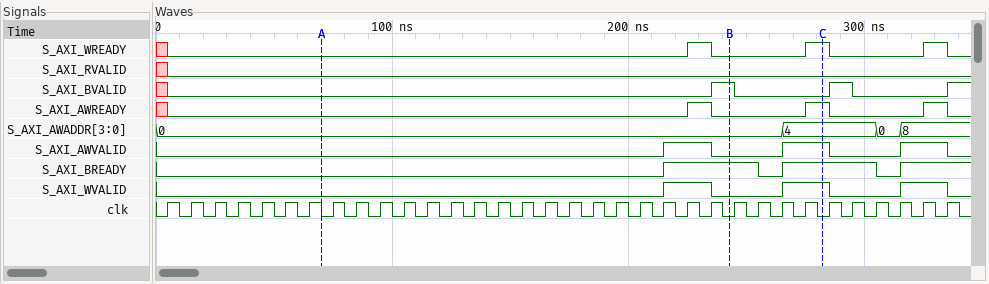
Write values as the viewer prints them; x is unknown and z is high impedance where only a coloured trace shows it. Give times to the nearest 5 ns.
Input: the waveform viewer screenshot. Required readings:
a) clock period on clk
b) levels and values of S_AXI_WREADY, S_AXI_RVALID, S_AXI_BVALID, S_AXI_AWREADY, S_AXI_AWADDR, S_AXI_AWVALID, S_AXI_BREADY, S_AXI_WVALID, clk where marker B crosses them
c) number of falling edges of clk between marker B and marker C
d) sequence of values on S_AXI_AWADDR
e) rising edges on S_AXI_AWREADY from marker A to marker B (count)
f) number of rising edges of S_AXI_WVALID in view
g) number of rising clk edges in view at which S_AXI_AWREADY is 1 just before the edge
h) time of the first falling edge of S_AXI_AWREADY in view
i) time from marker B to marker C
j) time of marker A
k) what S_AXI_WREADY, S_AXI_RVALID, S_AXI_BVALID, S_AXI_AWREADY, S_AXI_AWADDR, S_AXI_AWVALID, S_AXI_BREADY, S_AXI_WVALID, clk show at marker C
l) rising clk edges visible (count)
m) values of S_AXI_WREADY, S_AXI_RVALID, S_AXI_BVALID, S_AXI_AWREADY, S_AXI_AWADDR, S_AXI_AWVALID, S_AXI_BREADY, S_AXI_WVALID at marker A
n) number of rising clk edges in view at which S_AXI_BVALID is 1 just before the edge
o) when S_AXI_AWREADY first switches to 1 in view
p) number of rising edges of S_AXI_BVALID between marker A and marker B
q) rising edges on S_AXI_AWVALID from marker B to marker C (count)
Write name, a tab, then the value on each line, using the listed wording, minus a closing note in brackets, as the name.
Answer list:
clock period on clk	10 ns
levels and values of S_AXI_WREADY, S_AXI_RVALID, S_AXI_BVALID, S_AXI_AWREADY, S_AXI_AWADDR, S_AXI_AWVALID, S_AXI_BREADY, S_AXI_WVALID, clk where marker B crosses them	S_AXI_WREADY=0, S_AXI_RVALID=0, S_AXI_BVALID=1, S_AXI_AWREADY=0, S_AXI_AWADDR=0, S_AXI_AWVALID=0, S_AXI_BREADY=1, S_AXI_WVALID=0, clk=0
number of falling edges of clk between marker B and marker C	4
sequence of values on S_AXI_AWADDR	0, 4, 0, 8
rising edges on S_AXI_AWREADY from marker A to marker B	1
number of rising edges of S_AXI_WVALID in view	3
number of rising clk edges in view at which S_AXI_AWREADY is 1 just before the edge	3
time of the first falling edge of S_AXI_AWREADY in view	235 ns
time from marker B to marker C	40 ns
time of marker A	70 ns
what S_AXI_WREADY, S_AXI_RVALID, S_AXI_BVALID, S_AXI_AWREADY, S_AXI_AWADDR, S_AXI_AWVALID, S_AXI_BREADY, S_AXI_WVALID, clk show at marker C	S_AXI_WREADY=1, S_AXI_RVALID=0, S_AXI_BVALID=0, S_AXI_AWREADY=1, S_AXI_AWADDR=4, S_AXI_AWVALID=1, S_AXI_BREADY=1, S_AXI_WVALID=1, clk=0
rising clk edges visible	34
values of S_AXI_WREADY, S_AXI_RVALID, S_AXI_BVALID, S_AXI_AWREADY, S_AXI_AWADDR, S_AXI_AWVALID, S_AXI_BREADY, S_AXI_WVALID at marker A	S_AXI_WREADY=0, S_AXI_RVALID=0, S_AXI_BVALID=0, S_AXI_AWREADY=0, S_AXI_AWADDR=0, S_AXI_AWVALID=0, S_AXI_BREADY=0, S_AXI_WVALID=0
number of rising clk edges in view at which S_AXI_BVALID is 1 just before the edge	2
when S_AXI_AWREADY first switches to 1 in view	225 ns
number of rising edges of S_AXI_BVALID between marker A and marker B	1
rising edges on S_AXI_AWVALID from marker B to marker C	1
